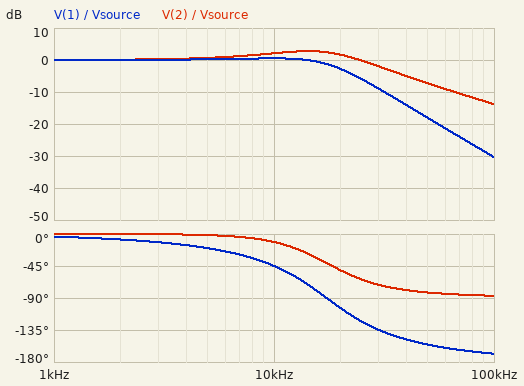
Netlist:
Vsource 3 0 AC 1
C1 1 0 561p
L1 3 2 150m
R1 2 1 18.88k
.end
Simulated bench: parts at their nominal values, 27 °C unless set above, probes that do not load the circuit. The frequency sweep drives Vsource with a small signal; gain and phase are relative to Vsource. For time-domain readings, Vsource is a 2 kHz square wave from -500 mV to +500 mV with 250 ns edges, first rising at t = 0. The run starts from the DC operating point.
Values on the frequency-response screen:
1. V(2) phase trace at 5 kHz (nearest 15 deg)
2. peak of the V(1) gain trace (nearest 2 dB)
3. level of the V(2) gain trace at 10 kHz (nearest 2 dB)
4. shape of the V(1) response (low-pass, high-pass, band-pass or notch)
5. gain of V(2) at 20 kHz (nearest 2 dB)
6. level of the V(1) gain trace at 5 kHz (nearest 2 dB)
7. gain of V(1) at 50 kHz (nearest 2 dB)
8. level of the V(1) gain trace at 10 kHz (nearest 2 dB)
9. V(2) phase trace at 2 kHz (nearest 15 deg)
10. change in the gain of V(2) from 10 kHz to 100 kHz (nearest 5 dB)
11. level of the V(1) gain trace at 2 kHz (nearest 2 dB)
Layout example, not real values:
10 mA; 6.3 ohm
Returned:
0 deg; 0 dB; 2 dB; low-pass; 2 dB; 0 dB; -18 dB; 0 dB; 0 deg; -15 dB; 0 dB
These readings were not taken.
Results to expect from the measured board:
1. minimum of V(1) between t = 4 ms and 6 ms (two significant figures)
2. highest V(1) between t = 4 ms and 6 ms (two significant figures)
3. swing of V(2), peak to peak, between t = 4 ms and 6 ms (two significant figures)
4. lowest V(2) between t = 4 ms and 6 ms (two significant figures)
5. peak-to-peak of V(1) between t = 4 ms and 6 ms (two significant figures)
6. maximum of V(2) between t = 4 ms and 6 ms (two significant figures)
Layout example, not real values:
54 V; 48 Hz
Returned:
-610 mV; 610 mV; 1.5 V; -760 mV; 1.2 V; 760 mV
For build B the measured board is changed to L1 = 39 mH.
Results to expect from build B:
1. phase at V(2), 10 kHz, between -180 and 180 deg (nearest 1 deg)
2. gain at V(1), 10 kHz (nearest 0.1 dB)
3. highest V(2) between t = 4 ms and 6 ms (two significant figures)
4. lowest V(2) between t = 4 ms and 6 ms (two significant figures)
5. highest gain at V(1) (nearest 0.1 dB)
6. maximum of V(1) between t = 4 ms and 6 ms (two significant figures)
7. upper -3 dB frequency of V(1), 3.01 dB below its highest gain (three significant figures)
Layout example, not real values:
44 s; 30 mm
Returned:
-2 deg; -1.1 dB; 620 mV; -620 mV; 0 dB; 500 mV; 18.4 kHz
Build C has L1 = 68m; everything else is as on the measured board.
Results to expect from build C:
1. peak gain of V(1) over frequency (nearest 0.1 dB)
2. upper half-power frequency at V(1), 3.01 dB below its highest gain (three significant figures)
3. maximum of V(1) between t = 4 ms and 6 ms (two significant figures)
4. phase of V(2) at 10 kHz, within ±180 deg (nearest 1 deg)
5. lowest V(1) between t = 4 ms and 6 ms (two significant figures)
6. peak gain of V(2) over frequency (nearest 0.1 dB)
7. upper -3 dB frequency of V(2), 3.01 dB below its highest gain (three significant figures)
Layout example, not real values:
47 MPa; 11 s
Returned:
0 dB; 20.5 kHz; 510 mV; -4 deg; -510 mV; 1.6 dB; 46.6 kHz
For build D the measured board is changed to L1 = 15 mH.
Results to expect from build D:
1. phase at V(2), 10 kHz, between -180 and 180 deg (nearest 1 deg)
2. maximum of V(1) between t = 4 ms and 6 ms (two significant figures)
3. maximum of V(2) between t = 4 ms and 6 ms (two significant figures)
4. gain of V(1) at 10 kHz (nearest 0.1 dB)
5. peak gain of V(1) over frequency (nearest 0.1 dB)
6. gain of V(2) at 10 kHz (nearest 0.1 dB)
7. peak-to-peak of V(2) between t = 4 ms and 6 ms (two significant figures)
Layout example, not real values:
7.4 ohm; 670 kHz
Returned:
-1 deg; 500 mV; 560 mV; -1.4 dB; 0 dB; 0.2 dB; 1.1 V
